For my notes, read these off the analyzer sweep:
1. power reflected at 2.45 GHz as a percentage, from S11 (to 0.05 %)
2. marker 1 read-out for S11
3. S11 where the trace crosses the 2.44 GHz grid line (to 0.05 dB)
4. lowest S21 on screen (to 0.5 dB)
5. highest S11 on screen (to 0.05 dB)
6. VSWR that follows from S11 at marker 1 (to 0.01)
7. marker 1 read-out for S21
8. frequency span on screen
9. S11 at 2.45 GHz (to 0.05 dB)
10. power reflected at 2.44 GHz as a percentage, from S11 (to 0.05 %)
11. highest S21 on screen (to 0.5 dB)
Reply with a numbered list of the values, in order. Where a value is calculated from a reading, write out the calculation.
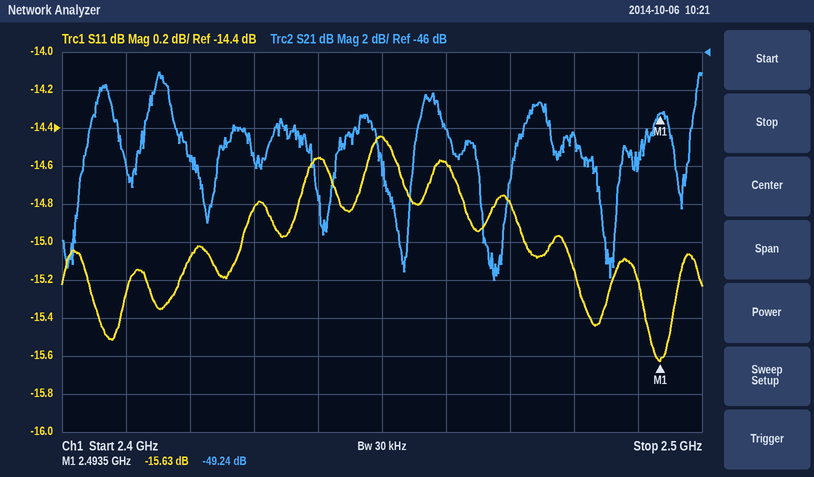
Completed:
1. 10^(-14.45/10) ≈ 3.59 %, so 3.60 % to the nearest 0.05 %
2. -15.63 dB
3. -14.55 dB
4. -58.0 dB
5. -14.45 dB
6. (1 + 0.1654)/(1 − 0.1654) ≈ 1.40
7. -49.24 dB
8. 100 MHz
9. -14.45 dB
10. 10^(-14.55/10) ≈ 3.51 %, so 3.50 % to the nearest 0.05 %
11. -47.0 dB
